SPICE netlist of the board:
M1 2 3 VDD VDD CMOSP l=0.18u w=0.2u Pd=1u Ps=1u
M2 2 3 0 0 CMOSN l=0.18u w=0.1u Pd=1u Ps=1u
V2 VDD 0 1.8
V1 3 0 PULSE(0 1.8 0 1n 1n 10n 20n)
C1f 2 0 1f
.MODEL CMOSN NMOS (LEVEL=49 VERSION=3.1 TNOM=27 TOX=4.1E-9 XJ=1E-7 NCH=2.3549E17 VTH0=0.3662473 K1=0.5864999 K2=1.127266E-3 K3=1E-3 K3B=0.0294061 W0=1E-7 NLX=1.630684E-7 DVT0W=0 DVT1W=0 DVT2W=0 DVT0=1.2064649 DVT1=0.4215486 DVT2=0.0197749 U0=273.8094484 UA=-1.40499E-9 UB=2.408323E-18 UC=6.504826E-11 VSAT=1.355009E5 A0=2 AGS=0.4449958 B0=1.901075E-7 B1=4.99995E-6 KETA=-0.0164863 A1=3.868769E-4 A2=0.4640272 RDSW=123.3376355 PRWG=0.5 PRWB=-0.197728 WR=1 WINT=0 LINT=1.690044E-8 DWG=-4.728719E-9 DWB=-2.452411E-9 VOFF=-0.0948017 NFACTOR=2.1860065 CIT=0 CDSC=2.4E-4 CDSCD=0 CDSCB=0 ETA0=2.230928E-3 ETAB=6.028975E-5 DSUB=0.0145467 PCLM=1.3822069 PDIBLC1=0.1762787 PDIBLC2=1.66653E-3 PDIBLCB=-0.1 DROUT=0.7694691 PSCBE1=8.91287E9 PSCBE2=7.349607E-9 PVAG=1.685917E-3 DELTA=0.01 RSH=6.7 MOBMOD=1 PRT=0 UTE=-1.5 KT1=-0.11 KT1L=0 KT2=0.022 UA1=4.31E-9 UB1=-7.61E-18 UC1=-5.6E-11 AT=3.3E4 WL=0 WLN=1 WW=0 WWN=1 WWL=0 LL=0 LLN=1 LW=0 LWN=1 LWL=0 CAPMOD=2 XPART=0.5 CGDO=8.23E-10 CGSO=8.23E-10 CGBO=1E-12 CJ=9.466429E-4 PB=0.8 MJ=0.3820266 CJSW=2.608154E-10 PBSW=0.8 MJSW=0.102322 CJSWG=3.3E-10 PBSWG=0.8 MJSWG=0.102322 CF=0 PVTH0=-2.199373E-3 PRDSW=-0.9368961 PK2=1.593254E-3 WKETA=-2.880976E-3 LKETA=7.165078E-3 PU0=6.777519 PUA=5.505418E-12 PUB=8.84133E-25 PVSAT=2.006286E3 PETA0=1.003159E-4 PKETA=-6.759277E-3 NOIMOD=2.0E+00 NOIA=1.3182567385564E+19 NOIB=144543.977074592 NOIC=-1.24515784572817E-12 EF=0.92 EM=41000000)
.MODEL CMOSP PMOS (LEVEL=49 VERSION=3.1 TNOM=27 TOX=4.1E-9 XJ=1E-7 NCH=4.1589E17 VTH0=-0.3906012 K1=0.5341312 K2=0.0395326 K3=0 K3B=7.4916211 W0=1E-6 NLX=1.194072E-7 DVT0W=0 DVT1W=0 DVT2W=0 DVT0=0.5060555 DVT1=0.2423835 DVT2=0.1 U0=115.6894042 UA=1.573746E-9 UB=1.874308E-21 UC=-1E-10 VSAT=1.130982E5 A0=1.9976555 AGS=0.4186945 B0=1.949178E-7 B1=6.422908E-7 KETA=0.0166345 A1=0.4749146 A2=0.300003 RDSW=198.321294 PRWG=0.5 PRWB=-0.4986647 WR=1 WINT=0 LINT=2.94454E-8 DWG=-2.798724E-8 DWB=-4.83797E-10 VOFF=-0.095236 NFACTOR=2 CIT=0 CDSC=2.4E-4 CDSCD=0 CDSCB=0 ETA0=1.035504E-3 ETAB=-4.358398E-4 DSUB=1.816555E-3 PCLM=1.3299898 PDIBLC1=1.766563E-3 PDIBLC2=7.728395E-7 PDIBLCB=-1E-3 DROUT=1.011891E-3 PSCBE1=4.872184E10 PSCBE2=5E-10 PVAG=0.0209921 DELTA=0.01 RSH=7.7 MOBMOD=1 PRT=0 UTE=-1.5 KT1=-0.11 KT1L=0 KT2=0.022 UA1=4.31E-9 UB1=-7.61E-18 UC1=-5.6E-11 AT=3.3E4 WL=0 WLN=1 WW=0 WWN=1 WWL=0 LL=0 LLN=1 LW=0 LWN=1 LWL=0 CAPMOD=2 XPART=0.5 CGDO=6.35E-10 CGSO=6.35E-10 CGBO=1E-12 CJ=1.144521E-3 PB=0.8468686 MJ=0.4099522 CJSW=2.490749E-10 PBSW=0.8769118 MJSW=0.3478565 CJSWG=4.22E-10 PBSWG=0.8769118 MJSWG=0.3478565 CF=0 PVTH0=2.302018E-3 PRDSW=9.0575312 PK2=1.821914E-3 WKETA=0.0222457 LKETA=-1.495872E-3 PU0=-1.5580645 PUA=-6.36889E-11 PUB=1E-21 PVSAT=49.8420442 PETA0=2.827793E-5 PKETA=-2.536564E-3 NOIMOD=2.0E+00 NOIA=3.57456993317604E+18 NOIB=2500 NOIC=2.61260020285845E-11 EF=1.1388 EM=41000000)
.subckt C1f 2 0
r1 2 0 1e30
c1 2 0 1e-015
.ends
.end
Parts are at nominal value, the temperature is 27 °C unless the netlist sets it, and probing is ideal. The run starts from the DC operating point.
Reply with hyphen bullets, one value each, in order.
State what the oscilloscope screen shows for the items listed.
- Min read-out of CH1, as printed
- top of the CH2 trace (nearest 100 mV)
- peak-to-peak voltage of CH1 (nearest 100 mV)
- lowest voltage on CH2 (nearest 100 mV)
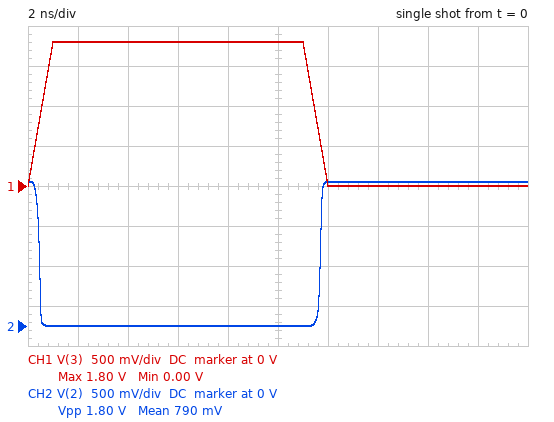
- 0.00 V
- 1.8 V
- 1.8 V
- 0 V
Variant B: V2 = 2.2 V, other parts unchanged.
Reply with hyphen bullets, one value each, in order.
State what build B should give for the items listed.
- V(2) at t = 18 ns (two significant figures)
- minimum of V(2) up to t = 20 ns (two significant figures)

- 2.2 V
- -1.1 mV
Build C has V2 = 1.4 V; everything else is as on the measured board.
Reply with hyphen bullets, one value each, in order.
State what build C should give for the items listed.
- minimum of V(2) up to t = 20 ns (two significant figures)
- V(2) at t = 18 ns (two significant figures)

- -1.9 mV
- 1.4 V
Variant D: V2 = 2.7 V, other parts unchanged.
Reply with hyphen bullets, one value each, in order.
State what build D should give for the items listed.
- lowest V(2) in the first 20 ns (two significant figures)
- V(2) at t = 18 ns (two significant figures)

- 37 mV
- 2.7 V
